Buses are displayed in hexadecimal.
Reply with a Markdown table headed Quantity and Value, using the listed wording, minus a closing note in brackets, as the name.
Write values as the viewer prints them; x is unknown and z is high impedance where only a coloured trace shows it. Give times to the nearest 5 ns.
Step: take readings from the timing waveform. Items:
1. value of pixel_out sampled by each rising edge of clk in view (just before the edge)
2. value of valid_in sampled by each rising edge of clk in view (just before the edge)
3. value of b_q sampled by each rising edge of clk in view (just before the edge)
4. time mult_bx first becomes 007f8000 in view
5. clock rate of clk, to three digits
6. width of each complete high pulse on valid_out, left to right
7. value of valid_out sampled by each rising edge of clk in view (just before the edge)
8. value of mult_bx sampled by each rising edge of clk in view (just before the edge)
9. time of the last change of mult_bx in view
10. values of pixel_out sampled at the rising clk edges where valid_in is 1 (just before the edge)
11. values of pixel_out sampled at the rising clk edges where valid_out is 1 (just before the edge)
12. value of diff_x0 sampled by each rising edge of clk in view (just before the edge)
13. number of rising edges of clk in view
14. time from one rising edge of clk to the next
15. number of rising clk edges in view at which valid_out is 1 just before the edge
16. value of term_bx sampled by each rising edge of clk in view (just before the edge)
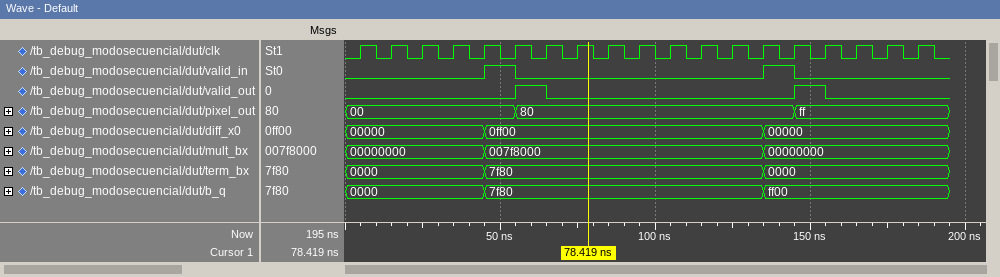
| Quantity | Value |
|---|---|
| value of pixel_out sampled by each rising edge of clk in view | 00, 00, 00, 00, 00, 00, 80, 80, 80, 80, 80, 80, 80, 80, 80, ff, ff, ff, ff |
| value of valid_in sampled by each rising edge of clk in view | 0 0 0 0 0 1 0 0 0 0 0 0 0 0 1 0 0 0 0 |
| value of b_q sampled by each rising edge of clk in view | 0000, 0000, 0000, 0000, 0000, 7f80, 7f80, 7f80, 7f80, 7f80, 7f80, 7f80, 7f80, 7f80, ff00, ff00, ff00, ff00, ff00 |
| time mult_bx first becomes 007f8000 in view | 45 ns |
| clock rate of clk, to three digits | 100 MHz |
| width of each complete high pulse on valid_out, left to right | 10 ns, 10 ns |
| value of valid_out sampled by each rising edge of clk in view | 0 0 0 0 0 0 1 0 0 0 0 0 0 0 0 1 0 0 0 |
| value of mult_bx sampled by each rising edge of clk in view | 00000000, 00000000, 00000000, 00000000, 00000000, 007f8000, 007f8000, 007f8000, 007f8000, 007f8000, 007f8000, 007f8000, 007f8000, 007f8000, 00000000, 00000000, 00000000, 00000000, 00000000 |
| time of the last change of mult_bx in view | 135 ns |
| values of pixel_out sampled at the rising clk edges where valid_in is 1 | 00, 80 |
| values of pixel_out sampled at the rising clk edges where valid_out is 1 | 80, ff |
| value of diff_x0 sampled by each rising edge of clk in view | 00000, 00000, 00000, 00000, 00000, 0ff00, 0ff00, 0ff00, 0ff00, 0ff00, 0ff00, 0ff00, 0ff00, 0ff00, 00000, 00000, 00000, 00000, 00000 |
| number of rising edges of clk in view | 19 |
| time from one rising edge of clk to the next | 10 ns |
| number of rising clk edges in view at which valid_out is 1 just before the edge | 2 |
| value of term_bx sampled by each rising edge of clk in view | 0000, 0000, 0000, 0000, 0000, 7f80, 7f80, 7f80, 7f80, 7f80, 7f80, 7f80, 7f80, 7f80, 0000, 0000, 0000, 0000, 0000 |
